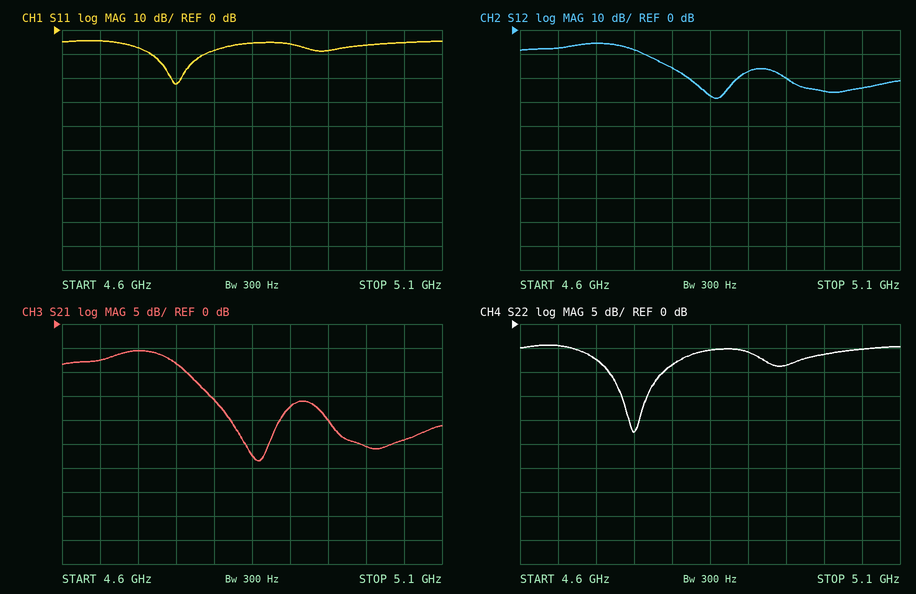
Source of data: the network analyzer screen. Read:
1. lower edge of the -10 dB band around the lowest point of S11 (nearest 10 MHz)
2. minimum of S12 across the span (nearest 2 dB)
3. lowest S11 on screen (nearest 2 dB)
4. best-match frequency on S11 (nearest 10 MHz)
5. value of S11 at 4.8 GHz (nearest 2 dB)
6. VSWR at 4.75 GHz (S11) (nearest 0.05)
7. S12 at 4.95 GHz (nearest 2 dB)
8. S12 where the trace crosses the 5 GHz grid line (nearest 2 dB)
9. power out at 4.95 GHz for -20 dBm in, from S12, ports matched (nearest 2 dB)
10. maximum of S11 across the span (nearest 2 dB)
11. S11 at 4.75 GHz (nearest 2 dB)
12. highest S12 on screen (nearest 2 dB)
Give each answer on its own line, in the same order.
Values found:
4.72 GHz
-28 dB
-22 dB
4.75 GHz
-8 dB
1.15
-20 dB
-26 dB
-40 dBm
-4 dB
-22 dB
-6 dB
